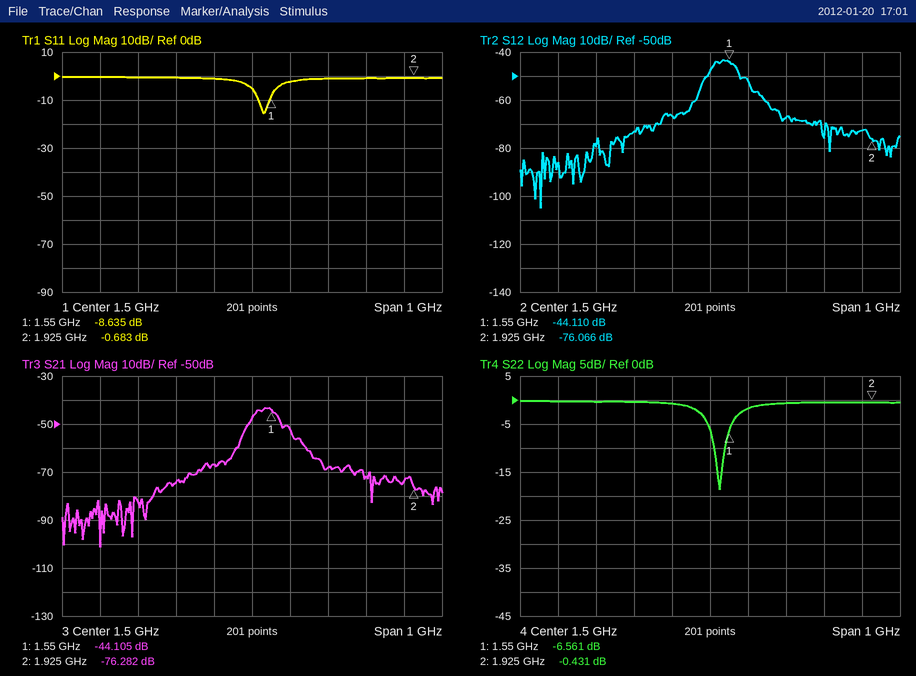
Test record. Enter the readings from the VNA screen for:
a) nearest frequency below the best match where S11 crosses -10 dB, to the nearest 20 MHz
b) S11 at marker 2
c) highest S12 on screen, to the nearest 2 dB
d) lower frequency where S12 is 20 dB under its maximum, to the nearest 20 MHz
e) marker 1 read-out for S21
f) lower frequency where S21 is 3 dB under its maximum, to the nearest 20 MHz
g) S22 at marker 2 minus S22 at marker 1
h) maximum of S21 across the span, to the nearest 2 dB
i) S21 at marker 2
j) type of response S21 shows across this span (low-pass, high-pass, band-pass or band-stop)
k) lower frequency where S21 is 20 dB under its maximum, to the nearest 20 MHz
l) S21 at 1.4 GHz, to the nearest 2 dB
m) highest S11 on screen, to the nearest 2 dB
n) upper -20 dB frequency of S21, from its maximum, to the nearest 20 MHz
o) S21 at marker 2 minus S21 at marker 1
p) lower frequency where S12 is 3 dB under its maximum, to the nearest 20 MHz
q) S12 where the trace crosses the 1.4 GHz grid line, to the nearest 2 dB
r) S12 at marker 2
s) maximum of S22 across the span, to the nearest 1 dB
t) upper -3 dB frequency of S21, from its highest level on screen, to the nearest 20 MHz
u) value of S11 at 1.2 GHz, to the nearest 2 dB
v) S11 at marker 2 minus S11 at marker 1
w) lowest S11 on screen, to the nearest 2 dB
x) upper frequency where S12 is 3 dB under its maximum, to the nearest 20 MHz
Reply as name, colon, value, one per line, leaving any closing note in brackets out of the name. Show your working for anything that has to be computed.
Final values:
nearest frequency below the best match where S11 crosses -10 dB, to the nearest 20 MHz: 1.52 GHz
S11 at marker 2: -0.683 dB
highest S12 on screen, to the nearest 2 dB: -44 dB
lower frequency where S12 is 20 dB under its maximum, to the nearest 20 MHz: 1.44 GHz
marker 1 read-out for S21: -44.105 dB
lower frequency where S21 is 3 dB under its maximum, to the nearest 20 MHz: 1.50 GHz
S22 at marker 2 minus S22 at marker 1: -0.431 − (-6.561) = 6.130 dB
maximum of S21 across the span, to the nearest 2 dB: -44 dB
S21 at marker 2: -76.282 dB
type of response S21 shows across this span: band-pass
lower frequency where S21 is 20 dB under its maximum, to the nearest 20 MHz: 1.44 GHz
S21 at 1.4 GHz, to the nearest 2 dB: -66 dB
highest S11 on screen, to the nearest 2 dB: 0 dB
upper -20 dB frequency of S21, from its maximum, to the nearest 20 MHz: 1.66 GHz
S21 at marker 2 minus S21 at marker 1: -76.282 − (-44.105) = -32.177 dB
lower frequency where S12 is 3 dB under its maximum, to the nearest 20 MHz: 1.50 GHz
S12 where the trace crosses the 1.4 GHz grid line, to the nearest 2 dB: -66 dB
S12 at marker 2: -76.066 dB
maximum of S22 across the span, to the nearest 1 dB: 0 dB
upper -3 dB frequency of S21, from its highest level on screen, to the nearest 20 MHz: 1.56 GHz
value of S11 at 1.2 GHz, to the nearest 2 dB: 0 dB
S11 at marker 2 minus S11 at marker 1: -0.683 − (-8.635) = 7.952 dB
lowest S11 on screen, to the nearest 2 dB: -16 dB
upper frequency where S12 is 3 dB under its maximum, to the nearest 20 MHz: 1.56 GHz
